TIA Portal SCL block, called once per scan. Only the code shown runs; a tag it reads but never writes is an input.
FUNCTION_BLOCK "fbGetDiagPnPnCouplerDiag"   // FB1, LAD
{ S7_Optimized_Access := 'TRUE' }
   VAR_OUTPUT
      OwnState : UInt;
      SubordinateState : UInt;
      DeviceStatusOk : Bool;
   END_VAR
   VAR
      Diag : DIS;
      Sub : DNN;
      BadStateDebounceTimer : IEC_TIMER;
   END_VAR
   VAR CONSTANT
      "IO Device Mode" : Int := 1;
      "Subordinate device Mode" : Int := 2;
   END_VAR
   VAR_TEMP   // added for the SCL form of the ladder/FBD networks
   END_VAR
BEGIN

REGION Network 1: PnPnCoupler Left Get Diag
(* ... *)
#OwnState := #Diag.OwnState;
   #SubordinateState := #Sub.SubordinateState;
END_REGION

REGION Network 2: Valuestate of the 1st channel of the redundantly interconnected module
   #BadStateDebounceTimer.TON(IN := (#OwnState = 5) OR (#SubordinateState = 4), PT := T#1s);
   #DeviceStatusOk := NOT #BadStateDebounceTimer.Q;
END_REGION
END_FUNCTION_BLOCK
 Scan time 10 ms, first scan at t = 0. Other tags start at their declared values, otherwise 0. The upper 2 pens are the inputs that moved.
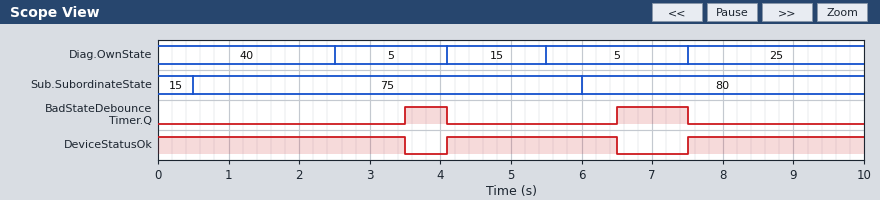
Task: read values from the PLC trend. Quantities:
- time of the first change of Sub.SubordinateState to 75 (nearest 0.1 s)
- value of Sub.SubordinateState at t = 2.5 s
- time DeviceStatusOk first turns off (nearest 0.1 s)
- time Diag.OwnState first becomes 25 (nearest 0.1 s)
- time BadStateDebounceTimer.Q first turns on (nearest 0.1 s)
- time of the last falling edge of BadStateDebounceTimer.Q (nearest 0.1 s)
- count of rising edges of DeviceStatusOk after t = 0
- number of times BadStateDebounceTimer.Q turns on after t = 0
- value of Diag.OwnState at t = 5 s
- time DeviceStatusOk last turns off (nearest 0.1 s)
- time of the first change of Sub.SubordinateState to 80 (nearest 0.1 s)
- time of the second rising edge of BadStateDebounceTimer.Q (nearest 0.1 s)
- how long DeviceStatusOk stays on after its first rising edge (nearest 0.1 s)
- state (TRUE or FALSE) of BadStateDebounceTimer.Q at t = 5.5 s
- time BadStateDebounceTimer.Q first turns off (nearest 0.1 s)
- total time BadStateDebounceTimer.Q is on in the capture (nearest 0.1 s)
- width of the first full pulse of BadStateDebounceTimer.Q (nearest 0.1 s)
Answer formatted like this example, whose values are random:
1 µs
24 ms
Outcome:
0.5 s
75
3.5 s
7.5 s
3.5 s
7.5 s
2
2
15
6.5 s
6.0 s
6.5 s
2.4 s
FALSE
4.1 s
1.6 s
0.6 s
